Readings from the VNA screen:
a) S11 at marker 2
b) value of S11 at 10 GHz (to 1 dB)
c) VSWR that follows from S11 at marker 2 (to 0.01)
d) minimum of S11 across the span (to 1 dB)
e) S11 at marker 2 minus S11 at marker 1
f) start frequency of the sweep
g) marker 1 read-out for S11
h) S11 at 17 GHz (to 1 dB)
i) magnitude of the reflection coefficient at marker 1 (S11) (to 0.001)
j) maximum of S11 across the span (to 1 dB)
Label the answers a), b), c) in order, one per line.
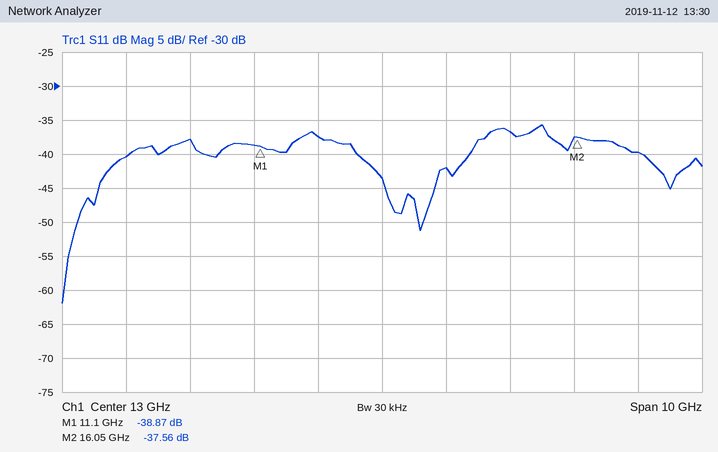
a) -37.56 dB
b) -38 dB
c) 1.03
d) -62 dB
e) 1.31 dB
f) 8 GHz
g) -38.87 dB
h) -40 dB
i) 0.011
j) -36 dB
